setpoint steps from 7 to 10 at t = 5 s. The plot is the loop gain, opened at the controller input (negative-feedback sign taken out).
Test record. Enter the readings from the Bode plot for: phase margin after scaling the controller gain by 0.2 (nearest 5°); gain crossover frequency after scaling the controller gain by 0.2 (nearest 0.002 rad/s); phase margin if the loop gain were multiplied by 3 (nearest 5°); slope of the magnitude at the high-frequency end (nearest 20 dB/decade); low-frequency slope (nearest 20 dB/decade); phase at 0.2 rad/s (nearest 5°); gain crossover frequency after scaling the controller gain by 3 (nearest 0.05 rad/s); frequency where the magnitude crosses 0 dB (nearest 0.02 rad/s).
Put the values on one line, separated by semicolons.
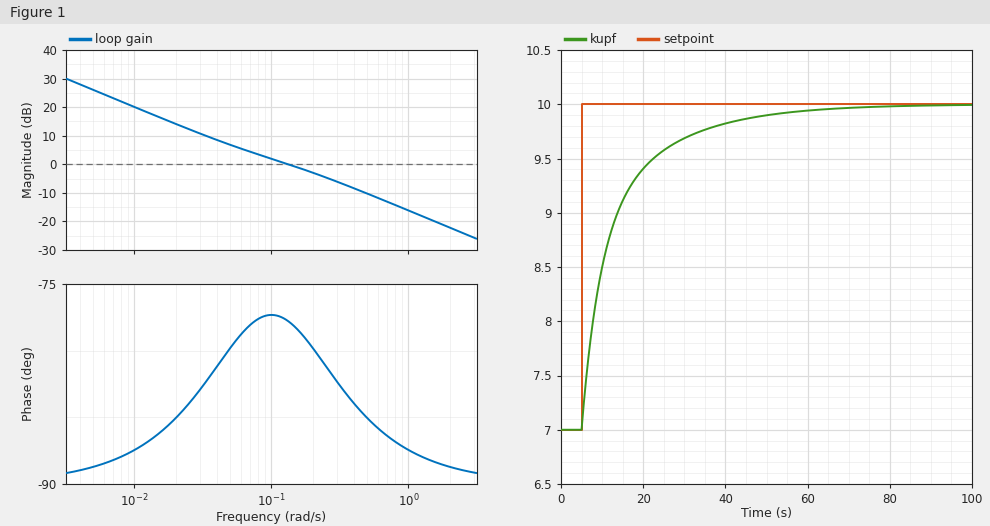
95°; 0.020 rad/s; 95°; -20 dB/decade; -20 dB/decade; -80°; 0.45 rad/s; 0.14 rad/s
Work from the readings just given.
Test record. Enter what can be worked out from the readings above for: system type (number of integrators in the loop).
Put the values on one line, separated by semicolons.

1
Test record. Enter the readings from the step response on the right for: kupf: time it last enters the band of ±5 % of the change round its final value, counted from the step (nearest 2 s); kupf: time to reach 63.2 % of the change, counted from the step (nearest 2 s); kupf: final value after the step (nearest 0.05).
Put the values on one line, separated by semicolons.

38 s; 8 s; 10.00
